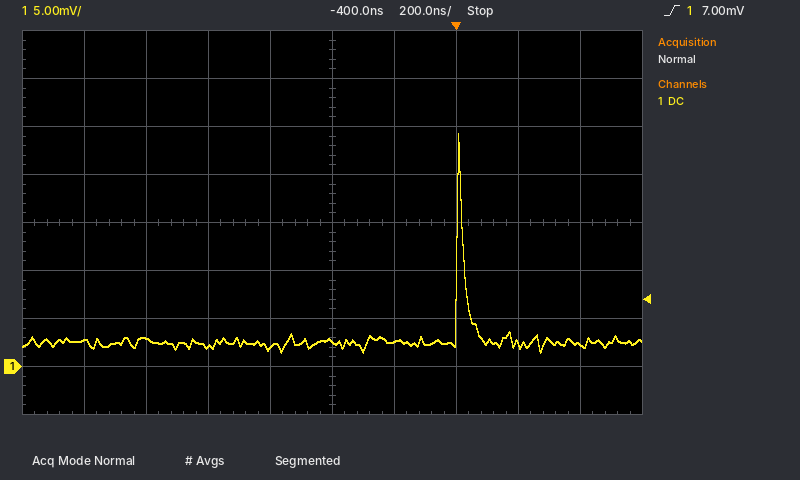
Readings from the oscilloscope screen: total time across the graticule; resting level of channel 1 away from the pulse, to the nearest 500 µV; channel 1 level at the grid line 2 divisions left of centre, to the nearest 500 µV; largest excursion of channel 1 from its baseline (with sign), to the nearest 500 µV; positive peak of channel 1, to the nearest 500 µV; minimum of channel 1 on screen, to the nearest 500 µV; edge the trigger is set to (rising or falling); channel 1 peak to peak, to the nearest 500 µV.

2 µs
2.5 mV
2.0 mV
+22.0 mV
24.5 mV
1.5 mV
rising
23.0 mV
